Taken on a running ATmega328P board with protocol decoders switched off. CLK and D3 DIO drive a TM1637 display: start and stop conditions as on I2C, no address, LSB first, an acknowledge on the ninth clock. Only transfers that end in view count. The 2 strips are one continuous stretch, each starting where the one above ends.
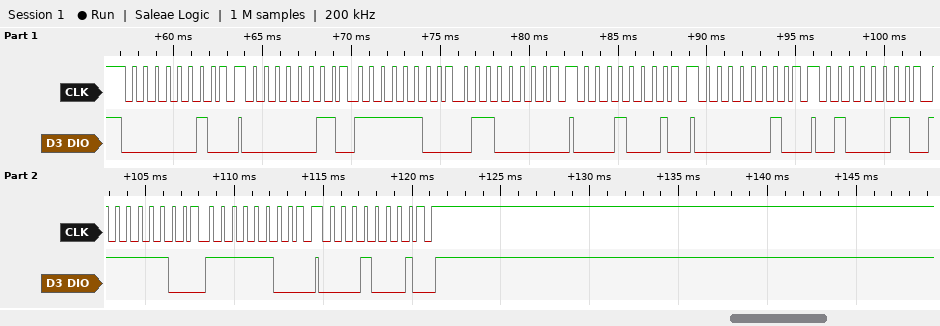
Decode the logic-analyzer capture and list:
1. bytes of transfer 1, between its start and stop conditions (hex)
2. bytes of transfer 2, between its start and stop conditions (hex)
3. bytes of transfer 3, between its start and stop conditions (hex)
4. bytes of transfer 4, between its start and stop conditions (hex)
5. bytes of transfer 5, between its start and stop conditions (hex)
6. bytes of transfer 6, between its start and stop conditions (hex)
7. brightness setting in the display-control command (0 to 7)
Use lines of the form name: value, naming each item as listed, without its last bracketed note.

bytes of transfer 1, between its start and stop conditions: 40
bytes of transfer 2, between its start and stop conditions: C0 3F 06
bytes of transfer 3, between its start and stop conditions: 88
bytes of transfer 4, between its start and stop conditions: 40
bytes of transfer 5, between its start and stop conditions: C2 3F 3F
bytes of transfer 6, between its start and stop conditions: 88
brightness setting in the display-control command: 0
